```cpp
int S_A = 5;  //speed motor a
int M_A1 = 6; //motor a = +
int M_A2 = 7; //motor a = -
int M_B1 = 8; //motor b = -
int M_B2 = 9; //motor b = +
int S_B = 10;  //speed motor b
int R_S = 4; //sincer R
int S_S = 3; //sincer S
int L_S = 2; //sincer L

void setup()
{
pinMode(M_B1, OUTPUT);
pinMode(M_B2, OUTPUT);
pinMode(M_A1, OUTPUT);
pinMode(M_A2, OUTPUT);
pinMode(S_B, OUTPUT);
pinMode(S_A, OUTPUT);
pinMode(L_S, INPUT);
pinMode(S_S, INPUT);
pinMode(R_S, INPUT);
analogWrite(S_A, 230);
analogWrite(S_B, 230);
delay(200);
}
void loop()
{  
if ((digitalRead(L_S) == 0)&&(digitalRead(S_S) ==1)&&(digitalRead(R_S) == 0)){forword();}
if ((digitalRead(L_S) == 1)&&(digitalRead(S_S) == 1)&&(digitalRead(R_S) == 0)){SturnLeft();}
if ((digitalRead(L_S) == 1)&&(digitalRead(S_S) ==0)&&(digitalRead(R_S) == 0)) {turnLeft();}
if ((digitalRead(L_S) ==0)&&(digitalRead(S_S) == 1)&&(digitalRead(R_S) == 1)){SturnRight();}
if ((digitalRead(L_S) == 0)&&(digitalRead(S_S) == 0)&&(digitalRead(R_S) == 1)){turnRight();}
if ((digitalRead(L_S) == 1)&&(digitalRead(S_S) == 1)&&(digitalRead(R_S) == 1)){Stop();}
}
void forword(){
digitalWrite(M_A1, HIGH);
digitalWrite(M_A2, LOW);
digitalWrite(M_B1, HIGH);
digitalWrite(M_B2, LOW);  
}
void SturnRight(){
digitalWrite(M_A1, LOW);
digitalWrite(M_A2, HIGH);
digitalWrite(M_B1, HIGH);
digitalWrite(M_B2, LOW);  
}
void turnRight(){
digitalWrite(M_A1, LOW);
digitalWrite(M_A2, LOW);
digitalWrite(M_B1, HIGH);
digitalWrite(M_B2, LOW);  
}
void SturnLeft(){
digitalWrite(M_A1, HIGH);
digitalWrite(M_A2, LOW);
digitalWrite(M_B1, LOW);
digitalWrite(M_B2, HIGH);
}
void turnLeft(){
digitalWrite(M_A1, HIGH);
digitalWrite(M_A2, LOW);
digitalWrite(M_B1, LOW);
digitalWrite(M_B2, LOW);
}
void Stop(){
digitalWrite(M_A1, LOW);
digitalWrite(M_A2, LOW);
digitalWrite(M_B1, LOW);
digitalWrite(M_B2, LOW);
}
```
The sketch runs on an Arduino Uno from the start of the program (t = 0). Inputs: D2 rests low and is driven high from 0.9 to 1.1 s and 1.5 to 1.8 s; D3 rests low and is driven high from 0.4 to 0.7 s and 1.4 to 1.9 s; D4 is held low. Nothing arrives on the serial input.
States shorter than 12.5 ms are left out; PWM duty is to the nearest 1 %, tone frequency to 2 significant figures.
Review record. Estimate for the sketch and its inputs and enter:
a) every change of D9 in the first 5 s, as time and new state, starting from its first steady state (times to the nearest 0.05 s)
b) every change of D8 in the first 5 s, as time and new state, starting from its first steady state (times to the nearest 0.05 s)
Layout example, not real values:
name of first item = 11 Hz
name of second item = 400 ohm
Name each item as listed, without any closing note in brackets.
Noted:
every change of D9 in the first 5 s, as time and new state, starting from its first steady state = 0 s low; 1.5 s high; 1.8 s low
every change of D8 in the first 5 s, as time and new state, starting from its first steady state = 0 s low; 0.4 s high; 0.9 s low; 1.4 s high; 1.5 s low; 1.8 s high
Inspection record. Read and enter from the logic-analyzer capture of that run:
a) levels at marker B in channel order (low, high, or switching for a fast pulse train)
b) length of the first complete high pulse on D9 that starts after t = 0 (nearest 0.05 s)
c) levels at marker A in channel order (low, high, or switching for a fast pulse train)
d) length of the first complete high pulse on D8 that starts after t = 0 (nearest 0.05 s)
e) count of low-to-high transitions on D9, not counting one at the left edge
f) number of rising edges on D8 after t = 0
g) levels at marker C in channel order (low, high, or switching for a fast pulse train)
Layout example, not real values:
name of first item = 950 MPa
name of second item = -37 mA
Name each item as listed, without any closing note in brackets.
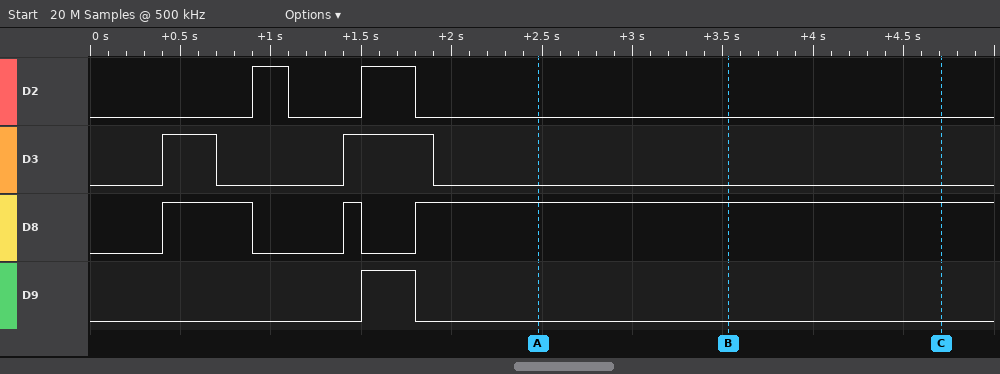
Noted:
levels at marker B in channel order = D2 low, D3 low, D8 high, D9 low
length of the first complete high pulse on D9 that starts after t = 0 = 0.30 s
levels at marker A in channel order = D2 low, D3 low, D8 high, D9 low
length of the first complete high pulse on D8 that starts after t = 0 = 0.50 s
count of low-to-high transitions on D9, not counting one at the left edge = 1
number of rising edges on D8 after t = 0 = 3
levels at marker C in channel order = D2 low, D3 low, D8 high, D9 low
